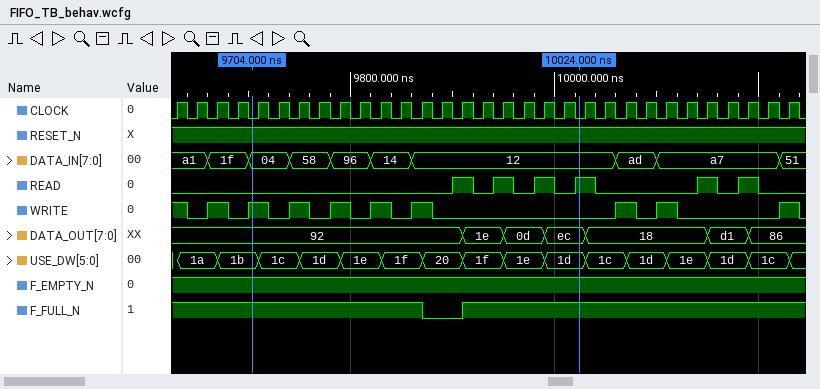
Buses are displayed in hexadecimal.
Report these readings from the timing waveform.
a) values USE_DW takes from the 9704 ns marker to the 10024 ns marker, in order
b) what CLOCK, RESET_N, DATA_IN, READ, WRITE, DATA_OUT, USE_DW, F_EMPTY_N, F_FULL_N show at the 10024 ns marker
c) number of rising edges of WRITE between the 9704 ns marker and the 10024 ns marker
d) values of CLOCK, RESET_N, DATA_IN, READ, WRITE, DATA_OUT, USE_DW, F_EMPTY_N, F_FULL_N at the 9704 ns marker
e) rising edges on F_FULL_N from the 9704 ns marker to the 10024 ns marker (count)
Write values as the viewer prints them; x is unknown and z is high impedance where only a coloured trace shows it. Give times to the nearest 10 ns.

1b, 1c, 1d, 1e, 1f, 20, 1f, 1e, 1d
CLOCK=0, RESET_N=1, DATA_IN=12, READ=1, WRITE=0, DATA_OUT=ec, USE_DW=1d, F_EMPTY_N=1, F_FULL_N=1
4
CLOCK=0, RESET_N=1, DATA_IN=04, READ=0, WRITE=1, DATA_OUT=92, USE_DW=1b, F_EMPTY_N=1, F_FULL_N=1
1
